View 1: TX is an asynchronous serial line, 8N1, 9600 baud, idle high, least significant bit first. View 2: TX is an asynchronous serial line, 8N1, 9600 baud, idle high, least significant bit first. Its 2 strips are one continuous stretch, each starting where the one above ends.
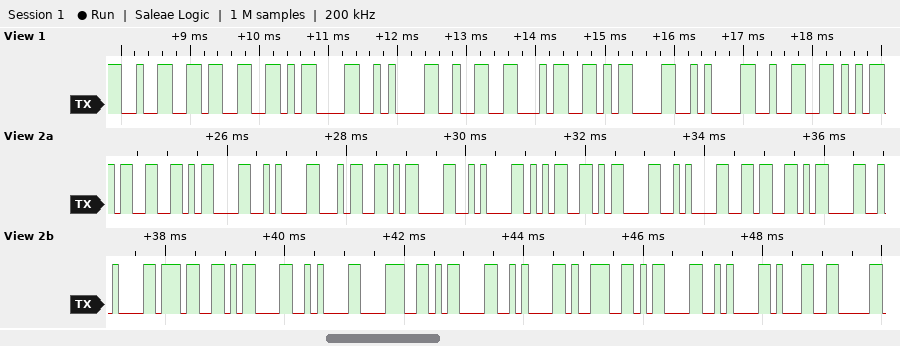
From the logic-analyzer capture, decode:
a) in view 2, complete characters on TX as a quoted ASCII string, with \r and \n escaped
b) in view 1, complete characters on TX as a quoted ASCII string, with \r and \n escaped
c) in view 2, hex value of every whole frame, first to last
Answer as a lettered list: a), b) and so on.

a) "3\r\n4\r\n5\r\n6\r\n7\r\n8\r\n9\r\n1"
b) "23\r\n24\r\n2"
c) 33 0D 0A 34 0D 0A 35 0D 0A 36 0D 0A 37 0D 0A 38 0D 0A 39 0D 0A 31
